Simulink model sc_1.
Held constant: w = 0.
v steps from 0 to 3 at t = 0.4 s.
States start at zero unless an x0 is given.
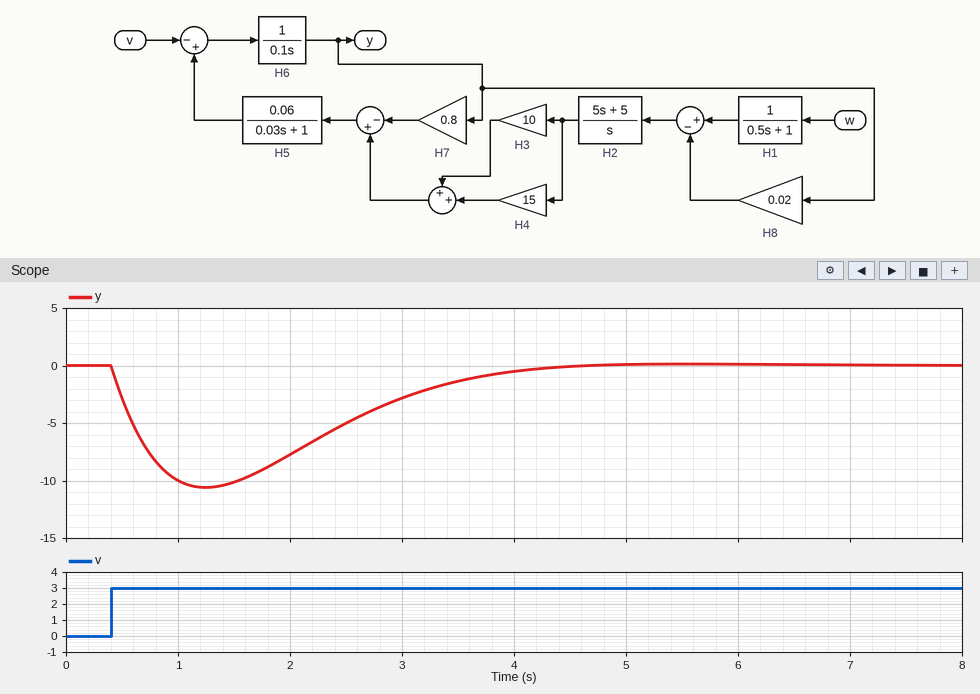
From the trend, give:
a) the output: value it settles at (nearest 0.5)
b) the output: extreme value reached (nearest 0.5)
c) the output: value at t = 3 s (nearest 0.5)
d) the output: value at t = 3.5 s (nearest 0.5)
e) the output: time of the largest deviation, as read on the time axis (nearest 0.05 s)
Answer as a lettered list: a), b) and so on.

a) 0.0
b) -10.5
c) -3.0
d) -1.5
e) 1.25 s
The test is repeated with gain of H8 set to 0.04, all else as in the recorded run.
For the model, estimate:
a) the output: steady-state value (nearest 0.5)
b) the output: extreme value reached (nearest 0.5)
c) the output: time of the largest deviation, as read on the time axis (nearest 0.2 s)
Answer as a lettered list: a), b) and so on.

a) 0.0
b) -6.5
c) 1.0 s
